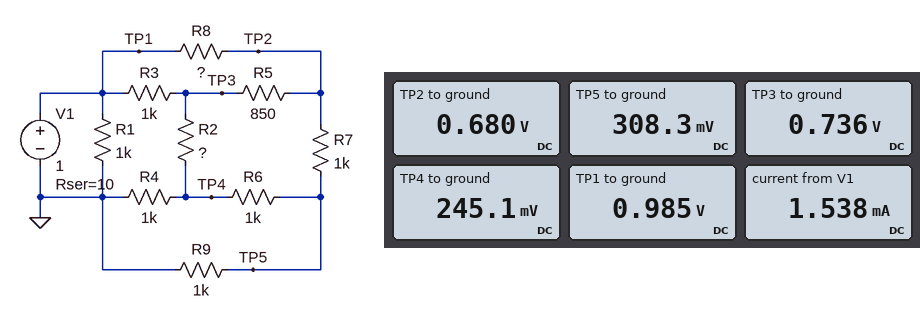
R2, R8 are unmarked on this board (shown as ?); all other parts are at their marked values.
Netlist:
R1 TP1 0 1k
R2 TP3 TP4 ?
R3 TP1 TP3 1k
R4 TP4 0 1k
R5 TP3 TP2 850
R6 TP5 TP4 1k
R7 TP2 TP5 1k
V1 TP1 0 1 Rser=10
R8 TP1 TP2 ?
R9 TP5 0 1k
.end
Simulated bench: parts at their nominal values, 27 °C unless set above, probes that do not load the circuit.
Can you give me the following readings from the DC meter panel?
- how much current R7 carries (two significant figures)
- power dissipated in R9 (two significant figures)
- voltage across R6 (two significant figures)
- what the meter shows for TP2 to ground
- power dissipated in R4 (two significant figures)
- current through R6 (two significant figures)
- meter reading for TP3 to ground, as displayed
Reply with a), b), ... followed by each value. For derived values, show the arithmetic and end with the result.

a) (680 mV - 308.3 mV) / 1 kΩ = 370 µA
b) (308.3 mV)^2 / 1 kΩ = 95 µW
c) 308.3 mV - 245.1 mV = 63 mV
d) 0.680 V
e) (245.1 mV)^2 / 1 kΩ = 60 µW
f) (308.3 mV - 245.1 mV) / 1 kΩ = 63 µA
g) 0.736 V
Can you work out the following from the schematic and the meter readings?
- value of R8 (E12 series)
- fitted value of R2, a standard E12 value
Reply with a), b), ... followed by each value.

a) 1 kΩ
b) 2.7 kΩ
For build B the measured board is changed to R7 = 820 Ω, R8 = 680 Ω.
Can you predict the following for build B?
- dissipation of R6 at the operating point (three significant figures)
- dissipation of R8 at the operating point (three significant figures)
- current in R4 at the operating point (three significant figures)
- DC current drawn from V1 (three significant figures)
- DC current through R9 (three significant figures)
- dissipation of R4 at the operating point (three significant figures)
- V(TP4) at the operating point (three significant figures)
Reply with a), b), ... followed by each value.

a) 7.52 µW
b) 106 µW
c) 268 µA
d) 1.61 mA
e) 354 µA
f) 71.6 µW
g) 268 mV
